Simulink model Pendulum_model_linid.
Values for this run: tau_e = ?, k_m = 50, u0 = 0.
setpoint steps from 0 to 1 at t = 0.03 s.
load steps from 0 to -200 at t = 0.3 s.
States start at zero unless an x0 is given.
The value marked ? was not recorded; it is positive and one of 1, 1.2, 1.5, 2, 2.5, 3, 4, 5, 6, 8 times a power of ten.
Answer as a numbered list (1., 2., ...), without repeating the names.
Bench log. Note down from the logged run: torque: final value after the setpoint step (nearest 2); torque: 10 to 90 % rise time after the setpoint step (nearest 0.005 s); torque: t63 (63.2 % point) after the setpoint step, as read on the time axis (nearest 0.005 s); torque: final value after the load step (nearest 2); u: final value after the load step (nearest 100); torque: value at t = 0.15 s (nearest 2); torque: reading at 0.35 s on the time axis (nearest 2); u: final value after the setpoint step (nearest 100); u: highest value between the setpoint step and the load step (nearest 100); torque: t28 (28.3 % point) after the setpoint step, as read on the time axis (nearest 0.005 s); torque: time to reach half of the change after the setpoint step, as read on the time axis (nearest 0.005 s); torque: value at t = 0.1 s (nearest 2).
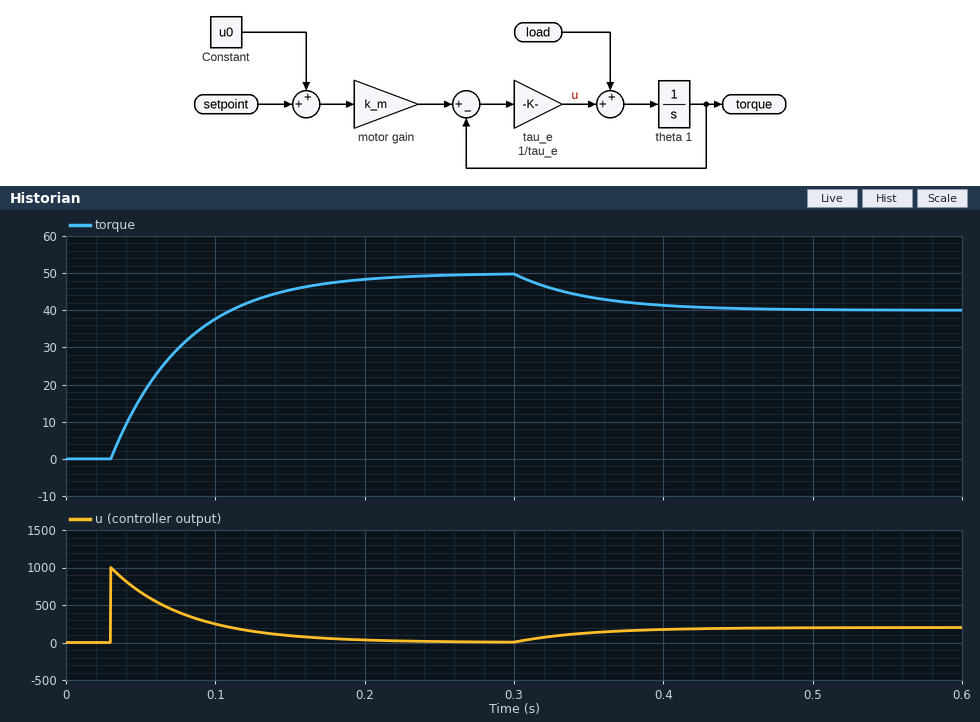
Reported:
1. 50
2. 0.110 s
3. 0.080 s
4. 40
5. 200
6. 46
7. 44
8. 0
9. 1000
10. 0.045 s
11. 0.065 s
12. 38
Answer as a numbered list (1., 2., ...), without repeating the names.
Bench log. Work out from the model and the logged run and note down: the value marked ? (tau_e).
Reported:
1. 0.05
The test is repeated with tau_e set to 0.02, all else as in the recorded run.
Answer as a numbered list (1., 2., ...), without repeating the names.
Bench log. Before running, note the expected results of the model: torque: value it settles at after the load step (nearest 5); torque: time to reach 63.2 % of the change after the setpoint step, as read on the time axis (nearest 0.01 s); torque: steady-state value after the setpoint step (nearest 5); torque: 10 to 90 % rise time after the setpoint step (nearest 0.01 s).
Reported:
1. 45
2. 0.05 s
3. 50
4. 0.04 s
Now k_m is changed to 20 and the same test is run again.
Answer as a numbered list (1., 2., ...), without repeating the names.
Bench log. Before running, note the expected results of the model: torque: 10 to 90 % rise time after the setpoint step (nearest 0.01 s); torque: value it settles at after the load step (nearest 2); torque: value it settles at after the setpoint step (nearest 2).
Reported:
1. 0.11 s
2. 10
3. 20
